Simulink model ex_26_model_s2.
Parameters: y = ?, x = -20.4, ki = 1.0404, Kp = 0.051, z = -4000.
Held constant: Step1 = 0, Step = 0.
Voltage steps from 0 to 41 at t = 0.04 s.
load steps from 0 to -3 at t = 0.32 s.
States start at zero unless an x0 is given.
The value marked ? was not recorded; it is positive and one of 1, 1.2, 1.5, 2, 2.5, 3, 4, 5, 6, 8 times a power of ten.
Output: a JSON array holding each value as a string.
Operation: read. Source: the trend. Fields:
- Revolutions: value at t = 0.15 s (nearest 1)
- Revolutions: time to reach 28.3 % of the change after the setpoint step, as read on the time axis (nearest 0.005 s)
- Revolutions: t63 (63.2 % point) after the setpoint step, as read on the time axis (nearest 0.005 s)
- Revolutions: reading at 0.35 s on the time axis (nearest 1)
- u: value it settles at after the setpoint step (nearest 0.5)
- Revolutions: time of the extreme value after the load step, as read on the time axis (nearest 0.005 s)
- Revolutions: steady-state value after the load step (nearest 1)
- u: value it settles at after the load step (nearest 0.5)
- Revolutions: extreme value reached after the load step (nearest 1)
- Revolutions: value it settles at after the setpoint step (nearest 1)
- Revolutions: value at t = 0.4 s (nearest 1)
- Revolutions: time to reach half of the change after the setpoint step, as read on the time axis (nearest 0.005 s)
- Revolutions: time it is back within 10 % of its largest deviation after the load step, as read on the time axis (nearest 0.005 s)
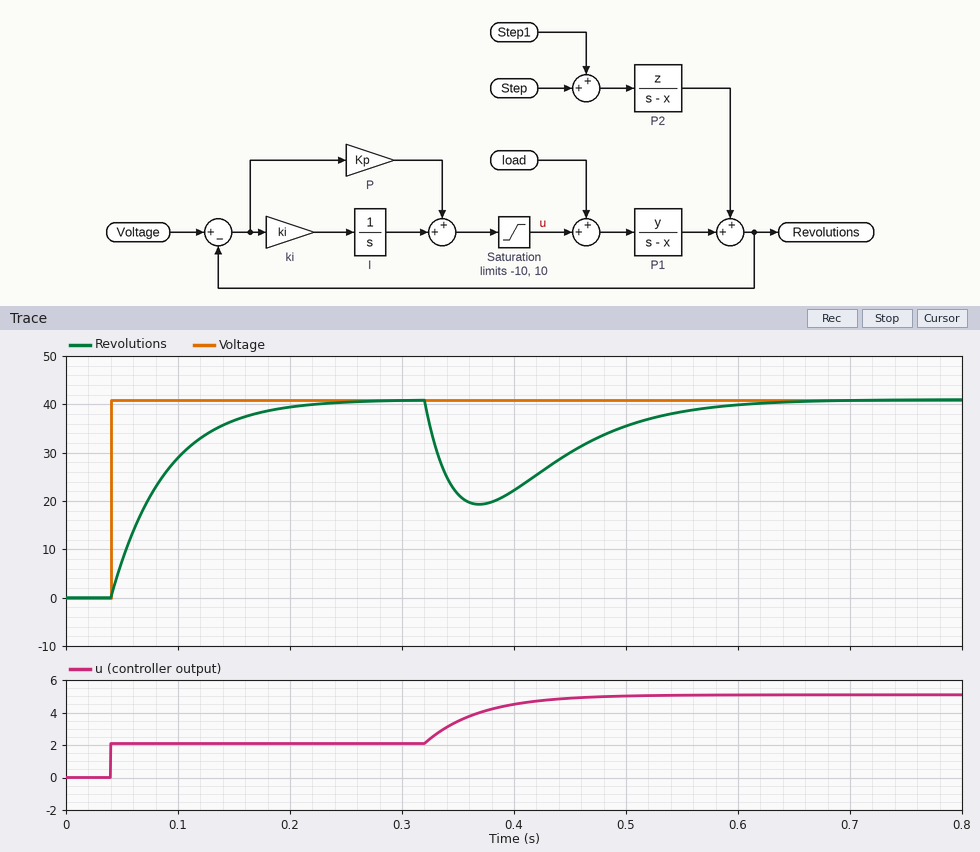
["37", "0.055 s", "0.090 s", "21", "2.0", "0.370 s", "41", "5.0", "19", "41", "22", "0.075 s", "0.560 s"]
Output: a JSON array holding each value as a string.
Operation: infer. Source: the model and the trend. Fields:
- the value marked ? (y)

["400"]
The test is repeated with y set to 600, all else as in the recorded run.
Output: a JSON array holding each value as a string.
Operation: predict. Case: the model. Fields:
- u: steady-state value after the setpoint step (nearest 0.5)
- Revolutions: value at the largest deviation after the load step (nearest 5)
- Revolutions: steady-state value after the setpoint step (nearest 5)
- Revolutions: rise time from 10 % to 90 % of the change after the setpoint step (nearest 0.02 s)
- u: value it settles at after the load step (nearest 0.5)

["1.5", "15", "40", "0.08 s", "4.5"]
